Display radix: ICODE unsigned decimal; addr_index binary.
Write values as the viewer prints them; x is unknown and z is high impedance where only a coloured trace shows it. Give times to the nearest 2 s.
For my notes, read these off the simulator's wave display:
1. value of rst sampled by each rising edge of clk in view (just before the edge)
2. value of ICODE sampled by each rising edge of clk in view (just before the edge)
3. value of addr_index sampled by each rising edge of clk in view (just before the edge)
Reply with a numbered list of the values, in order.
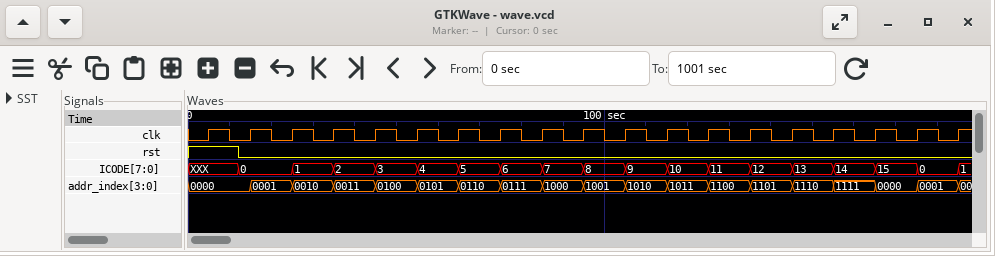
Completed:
1. 1 0 0 0 0 0 0 0 0 0 0 0 0 0 0 0 0 0 0
2. XXX, 0, 0, 1, 2, 3, 4, 5, 6, 7, 8, 9, 10, 11, 12, 13, 14, 15, 0
3. 0000, 0000, 0001, 0010, 0011, 0100, 0101, 0110, 0111, 1000, 1001, 1010, 1011, 1100, 1101, 1110, 1111, 0000, 0001
